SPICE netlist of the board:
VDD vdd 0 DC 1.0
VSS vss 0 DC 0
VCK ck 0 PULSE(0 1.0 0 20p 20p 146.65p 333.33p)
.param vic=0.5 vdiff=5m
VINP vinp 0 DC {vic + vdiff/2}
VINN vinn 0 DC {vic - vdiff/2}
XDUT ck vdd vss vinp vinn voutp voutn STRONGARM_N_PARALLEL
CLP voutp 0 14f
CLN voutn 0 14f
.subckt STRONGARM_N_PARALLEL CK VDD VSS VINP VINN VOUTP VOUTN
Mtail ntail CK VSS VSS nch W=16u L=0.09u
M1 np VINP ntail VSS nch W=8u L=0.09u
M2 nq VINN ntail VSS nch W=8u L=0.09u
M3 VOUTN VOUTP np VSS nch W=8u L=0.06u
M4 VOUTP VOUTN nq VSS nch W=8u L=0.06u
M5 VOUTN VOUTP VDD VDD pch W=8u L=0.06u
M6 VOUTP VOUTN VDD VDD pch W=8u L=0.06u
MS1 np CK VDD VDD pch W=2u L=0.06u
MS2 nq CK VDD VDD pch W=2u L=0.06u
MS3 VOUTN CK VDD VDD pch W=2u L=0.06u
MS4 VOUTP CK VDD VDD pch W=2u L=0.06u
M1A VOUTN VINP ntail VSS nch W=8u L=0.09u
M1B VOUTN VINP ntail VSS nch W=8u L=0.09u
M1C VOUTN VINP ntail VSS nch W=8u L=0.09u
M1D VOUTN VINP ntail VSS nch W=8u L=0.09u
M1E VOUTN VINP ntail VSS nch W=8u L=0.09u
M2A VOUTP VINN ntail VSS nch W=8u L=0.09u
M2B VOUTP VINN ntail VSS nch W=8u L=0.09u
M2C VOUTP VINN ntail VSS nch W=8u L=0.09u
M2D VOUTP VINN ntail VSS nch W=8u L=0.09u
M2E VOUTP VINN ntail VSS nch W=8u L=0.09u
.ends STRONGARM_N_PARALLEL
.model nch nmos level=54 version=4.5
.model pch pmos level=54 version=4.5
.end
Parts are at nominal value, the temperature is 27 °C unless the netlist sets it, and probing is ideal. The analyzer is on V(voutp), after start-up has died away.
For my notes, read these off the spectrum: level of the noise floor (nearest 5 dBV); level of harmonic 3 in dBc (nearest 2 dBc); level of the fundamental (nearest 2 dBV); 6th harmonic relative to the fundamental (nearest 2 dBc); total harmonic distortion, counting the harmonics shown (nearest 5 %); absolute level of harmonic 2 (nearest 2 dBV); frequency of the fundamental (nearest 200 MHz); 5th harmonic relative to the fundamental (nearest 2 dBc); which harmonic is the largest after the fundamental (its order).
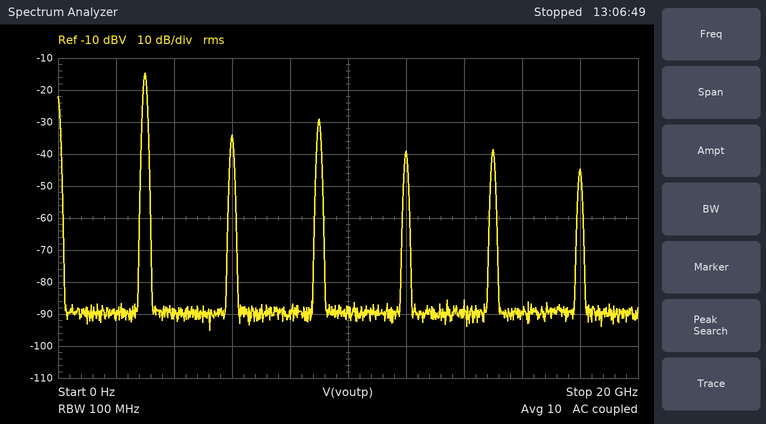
-90 dBV
-14 dBc
-14 dBV
-30 dBc
25 %
-34 dBV
3.0 GHz
-24 dBc
3
